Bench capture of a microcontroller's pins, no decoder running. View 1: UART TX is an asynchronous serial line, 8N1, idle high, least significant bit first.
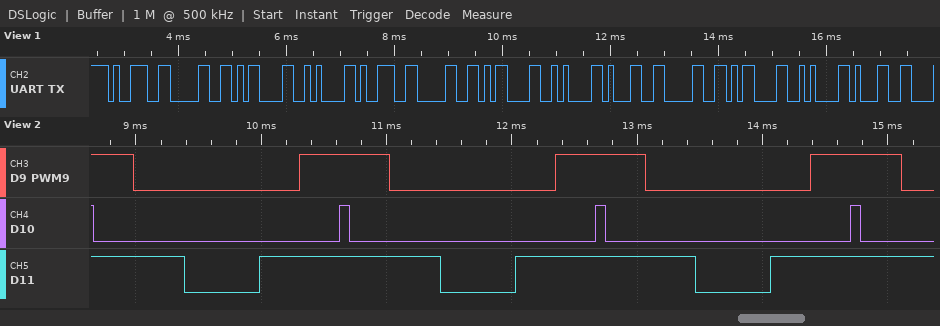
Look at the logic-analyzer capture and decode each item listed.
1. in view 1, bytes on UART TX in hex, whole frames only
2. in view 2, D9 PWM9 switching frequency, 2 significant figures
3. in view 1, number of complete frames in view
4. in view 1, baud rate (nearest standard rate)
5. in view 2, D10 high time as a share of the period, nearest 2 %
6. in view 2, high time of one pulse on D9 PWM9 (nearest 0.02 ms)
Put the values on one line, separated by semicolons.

39 30 0D 0A 39 30 0D 0A 31 30 0D 0A 31; 490 Hz; 13; 9600 baud; 4 %; 0.72 ms
